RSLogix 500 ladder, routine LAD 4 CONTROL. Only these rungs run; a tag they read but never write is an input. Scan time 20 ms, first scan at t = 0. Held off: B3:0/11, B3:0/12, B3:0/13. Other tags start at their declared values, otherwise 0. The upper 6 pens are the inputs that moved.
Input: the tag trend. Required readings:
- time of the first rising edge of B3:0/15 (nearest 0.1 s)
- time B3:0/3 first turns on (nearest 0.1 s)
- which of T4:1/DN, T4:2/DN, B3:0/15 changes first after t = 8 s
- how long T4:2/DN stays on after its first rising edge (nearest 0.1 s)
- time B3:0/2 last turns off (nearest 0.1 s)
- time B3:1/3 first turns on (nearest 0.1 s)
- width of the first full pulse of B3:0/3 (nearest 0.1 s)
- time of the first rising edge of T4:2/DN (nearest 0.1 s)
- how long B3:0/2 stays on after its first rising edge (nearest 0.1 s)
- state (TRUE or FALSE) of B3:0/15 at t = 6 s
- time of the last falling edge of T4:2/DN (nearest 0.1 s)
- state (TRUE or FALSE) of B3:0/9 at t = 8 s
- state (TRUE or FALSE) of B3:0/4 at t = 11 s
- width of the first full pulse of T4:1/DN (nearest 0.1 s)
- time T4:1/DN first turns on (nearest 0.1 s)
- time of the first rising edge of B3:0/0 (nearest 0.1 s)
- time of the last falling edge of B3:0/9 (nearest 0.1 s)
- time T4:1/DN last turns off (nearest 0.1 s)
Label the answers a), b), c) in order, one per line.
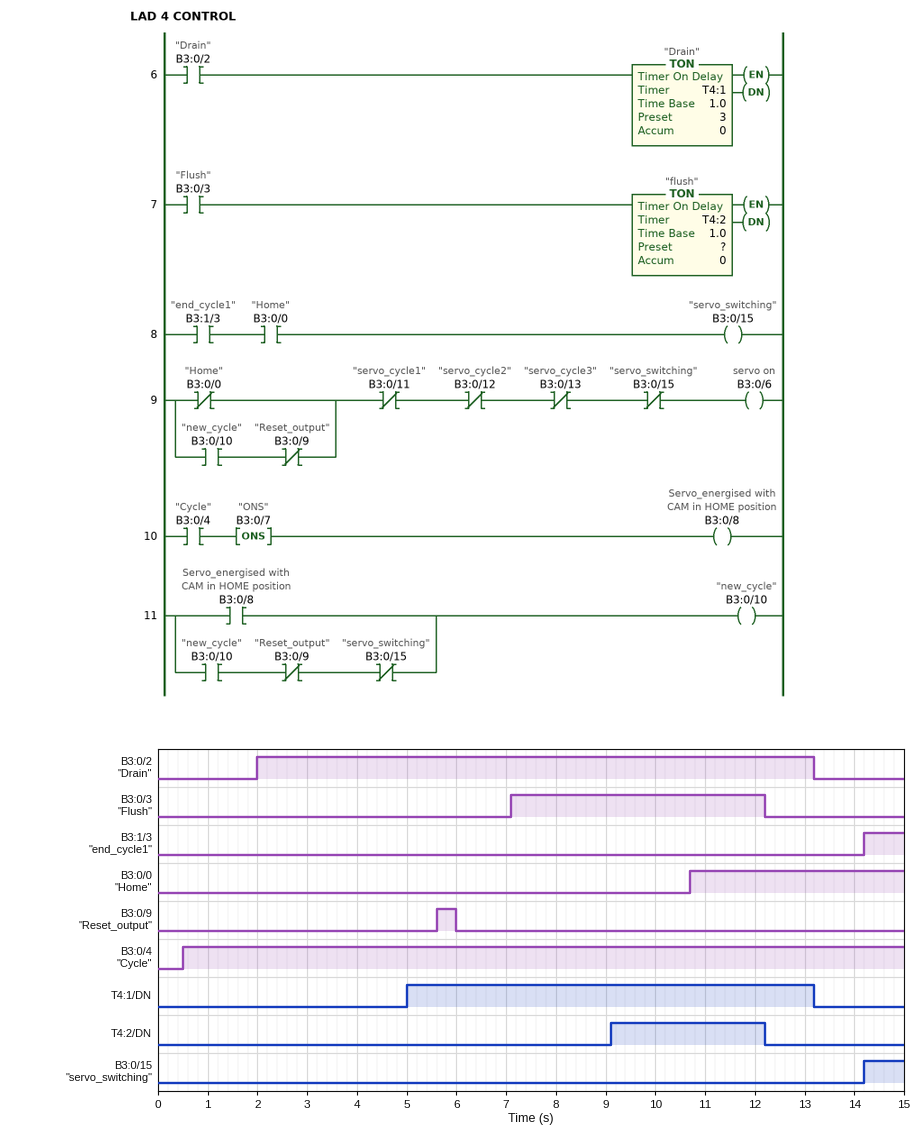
a) 14.2 s
b) 7.1 s
c) T4:2/DN
d) 3.1 s
e) 13.2 s
f) 14.2 s
g) 5.1 s
h) 9.1 s
i) 11.2 s
j) FALSE
k) 12.2 s
l) FALSE
m) TRUE
n) 8.2 s
o) 5.0 s
p) 10.7 s
q) 6.0 s
r) 13.2 s
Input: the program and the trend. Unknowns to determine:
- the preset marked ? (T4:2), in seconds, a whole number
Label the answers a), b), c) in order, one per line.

a) 2 s
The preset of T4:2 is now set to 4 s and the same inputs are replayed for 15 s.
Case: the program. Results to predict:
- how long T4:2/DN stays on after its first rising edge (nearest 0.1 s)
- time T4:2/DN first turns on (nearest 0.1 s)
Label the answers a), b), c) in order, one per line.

a) 1.1 s
b) 11.1 s
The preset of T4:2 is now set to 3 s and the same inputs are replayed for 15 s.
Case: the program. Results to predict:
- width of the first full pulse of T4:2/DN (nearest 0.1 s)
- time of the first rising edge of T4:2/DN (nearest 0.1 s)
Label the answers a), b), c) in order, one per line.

a) 2.1 s
b) 10.1 s
